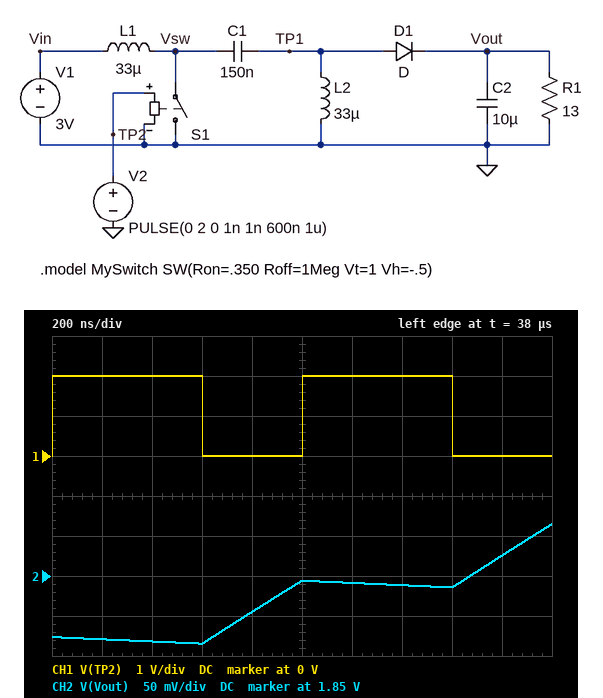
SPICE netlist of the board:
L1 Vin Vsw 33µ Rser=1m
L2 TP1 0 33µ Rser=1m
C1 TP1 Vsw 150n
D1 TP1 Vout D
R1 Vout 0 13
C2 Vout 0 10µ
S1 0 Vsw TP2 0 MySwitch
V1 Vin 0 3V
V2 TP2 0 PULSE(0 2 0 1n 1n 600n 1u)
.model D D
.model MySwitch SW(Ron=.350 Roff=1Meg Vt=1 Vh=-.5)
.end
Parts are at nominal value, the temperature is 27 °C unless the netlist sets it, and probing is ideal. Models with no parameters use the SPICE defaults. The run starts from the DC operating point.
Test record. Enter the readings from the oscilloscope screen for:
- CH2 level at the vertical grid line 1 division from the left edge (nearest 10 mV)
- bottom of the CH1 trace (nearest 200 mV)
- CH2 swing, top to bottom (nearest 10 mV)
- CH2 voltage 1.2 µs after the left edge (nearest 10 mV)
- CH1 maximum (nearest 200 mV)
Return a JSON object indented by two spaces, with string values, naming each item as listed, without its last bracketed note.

{
  "CH2 level at the vertical grid line 1 division from the left edge": "1.77 V",
  "bottom of the CH1 trace": "0 V",
  "CH2 swing, top to bottom": "150 mV",
  "CH2 voltage 1.2 µs after the left edge": "1.84 V",
  "CH1 maximum": "2.0 V"
}
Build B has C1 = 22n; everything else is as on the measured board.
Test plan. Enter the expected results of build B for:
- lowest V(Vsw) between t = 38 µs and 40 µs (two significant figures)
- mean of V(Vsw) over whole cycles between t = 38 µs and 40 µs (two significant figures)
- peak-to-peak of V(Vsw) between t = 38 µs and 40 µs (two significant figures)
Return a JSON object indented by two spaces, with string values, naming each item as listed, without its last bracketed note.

{
  "lowest V(Vsw) between t = 38 µs and 40 µs": "250 mV",
  "mean of V(Vsw) over whole cycles between t = 38 µs and 40 µs": "3.0 V",
  "peak-to-peak of V(Vsw) between t = 38 µs and 40 µs": "13 V"
}
